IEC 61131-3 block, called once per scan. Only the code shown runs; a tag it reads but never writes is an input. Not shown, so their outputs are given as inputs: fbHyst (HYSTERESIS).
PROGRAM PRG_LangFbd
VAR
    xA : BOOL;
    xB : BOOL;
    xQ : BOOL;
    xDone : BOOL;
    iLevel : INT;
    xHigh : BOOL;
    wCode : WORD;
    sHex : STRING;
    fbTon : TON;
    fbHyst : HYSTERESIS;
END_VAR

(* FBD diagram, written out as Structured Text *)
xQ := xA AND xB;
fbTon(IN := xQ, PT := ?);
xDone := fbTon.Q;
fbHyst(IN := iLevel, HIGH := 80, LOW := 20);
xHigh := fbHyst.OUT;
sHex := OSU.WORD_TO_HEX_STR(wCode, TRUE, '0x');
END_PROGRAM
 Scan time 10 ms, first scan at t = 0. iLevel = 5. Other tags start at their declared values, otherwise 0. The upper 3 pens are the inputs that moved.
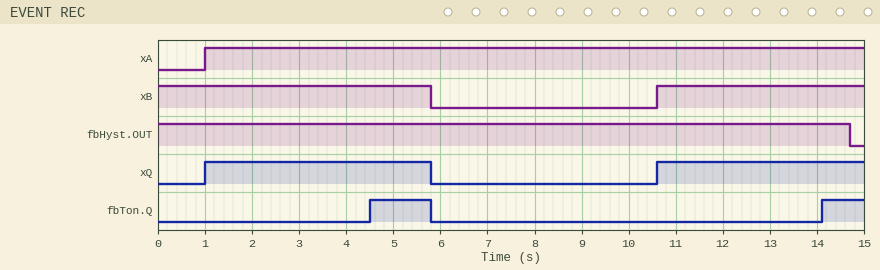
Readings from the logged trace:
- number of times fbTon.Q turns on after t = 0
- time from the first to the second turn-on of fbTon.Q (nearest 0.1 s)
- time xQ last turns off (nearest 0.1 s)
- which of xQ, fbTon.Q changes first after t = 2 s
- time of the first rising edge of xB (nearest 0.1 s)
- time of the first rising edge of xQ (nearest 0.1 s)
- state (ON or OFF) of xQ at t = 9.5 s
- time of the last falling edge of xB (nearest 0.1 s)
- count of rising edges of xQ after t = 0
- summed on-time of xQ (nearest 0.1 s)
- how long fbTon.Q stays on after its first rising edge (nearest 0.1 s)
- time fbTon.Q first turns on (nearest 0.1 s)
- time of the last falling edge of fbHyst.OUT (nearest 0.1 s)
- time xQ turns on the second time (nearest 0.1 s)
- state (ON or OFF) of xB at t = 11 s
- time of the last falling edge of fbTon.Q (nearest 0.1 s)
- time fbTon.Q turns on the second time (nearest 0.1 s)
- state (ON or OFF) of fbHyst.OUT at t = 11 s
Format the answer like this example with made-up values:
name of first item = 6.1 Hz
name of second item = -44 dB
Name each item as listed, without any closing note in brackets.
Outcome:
number of times fbTon.Q turns on after t = 0 = 2
time from the first to the second turn-on of fbTon.Q = 9.6 s
time xQ last turns off = 5.8 s
which of xQ, fbTon.Q changes first after t = 2 s = fbTon.Q
time of the first rising edge of xB = 10.6 s
time of the first rising edge of xQ = 1.0 s
state (ON or OFF) of xQ at t = 9.5 s = OFF
time of the last falling edge of xB = 5.8 s
count of rising edges of xQ after t = 0 = 2
summed on-time of xQ = 9.2 s
how long fbTon.Q stays on after its first rising edge = 1.3 s
time fbTon.Q first turns on = 4.5 s
time of the last falling edge of fbHyst.OUT = 14.7 s
time xQ turns on the second time = 10.6 s
state (ON or OFF) of xB at t = 11 s = ON
time of the last falling edge of fbTon.Q = 5.8 s
time fbTon.Q turns on the second time = 14.1 s
state (ON or OFF) of fbHyst.OUT at t = 11 s = ON
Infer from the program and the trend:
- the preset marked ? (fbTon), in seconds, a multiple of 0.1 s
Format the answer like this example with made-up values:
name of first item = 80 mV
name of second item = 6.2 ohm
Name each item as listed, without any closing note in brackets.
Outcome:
the preset marked ? (fbTon), in seconds, a multiple of 0.1 s = 3.5 s
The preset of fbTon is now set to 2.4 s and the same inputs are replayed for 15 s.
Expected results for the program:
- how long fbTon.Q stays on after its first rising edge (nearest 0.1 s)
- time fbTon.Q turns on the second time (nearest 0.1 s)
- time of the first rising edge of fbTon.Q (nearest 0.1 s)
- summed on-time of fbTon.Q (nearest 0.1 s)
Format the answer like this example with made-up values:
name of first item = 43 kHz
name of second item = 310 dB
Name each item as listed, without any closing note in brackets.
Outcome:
how long fbTon.Q stays on after its first rising edge = 2.4 s
time fbTon.Q turns on the second time = 13.0 s
time of the first rising edge of fbTon.Q = 3.4 s
summed on-time of fbTon.Q = 4.4 s
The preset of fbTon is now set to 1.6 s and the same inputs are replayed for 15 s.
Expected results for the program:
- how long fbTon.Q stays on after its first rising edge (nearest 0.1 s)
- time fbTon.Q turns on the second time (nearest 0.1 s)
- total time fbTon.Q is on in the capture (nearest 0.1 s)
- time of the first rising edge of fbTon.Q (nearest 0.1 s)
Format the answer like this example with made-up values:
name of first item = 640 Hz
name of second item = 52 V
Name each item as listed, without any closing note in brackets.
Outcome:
how long fbTon.Q stays on after its first rising edge = 3.2 s
time fbTon.Q turns on the second time = 12.2 s
total time fbTon.Q is on in the capture = 6.0 s
time of the first rising edge of fbTon.Q = 2.6 s
